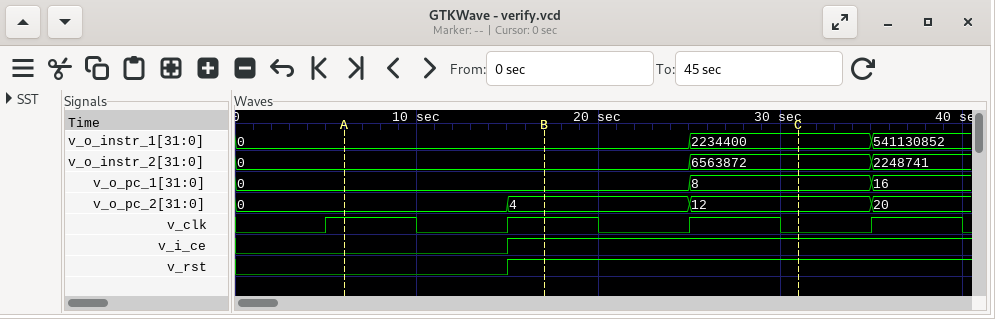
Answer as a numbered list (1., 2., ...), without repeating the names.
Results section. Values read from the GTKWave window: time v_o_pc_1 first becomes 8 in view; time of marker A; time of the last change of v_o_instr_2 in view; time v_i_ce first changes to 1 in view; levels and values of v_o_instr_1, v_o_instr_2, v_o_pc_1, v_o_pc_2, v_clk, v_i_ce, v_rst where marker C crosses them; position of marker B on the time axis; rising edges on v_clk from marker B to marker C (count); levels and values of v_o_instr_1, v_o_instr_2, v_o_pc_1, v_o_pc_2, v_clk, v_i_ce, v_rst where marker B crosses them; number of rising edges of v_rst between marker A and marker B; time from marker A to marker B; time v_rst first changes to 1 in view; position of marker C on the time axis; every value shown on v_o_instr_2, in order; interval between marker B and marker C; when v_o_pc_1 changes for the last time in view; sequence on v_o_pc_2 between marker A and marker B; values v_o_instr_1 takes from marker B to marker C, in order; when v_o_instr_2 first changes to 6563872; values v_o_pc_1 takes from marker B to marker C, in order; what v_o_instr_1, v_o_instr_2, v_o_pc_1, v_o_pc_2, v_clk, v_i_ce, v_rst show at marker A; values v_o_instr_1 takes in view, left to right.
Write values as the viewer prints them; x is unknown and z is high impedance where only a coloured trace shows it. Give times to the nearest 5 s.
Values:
1. 25 s
2. 5 s
3. 35 s
4. 15 s
5. v_o_instr_1=2234400, v_o_instr_2=6563872, v_o_pc_1=8, v_o_pc_2=12, v_clk=0, v_i_ce=1, v_rst=1
6. 15 s
7. 1
8. v_o_instr_1=0, v_o_instr_2=0, v_o_pc_1=0, v_o_pc_2=4, v_clk=1, v_i_ce=1, v_rst=1
9. 1
10. 10 s
11. 15 s
12. 30 s
13. 0, 6563872, 2248741
14. 15 s
15. 35 s
16. 0, 4
17. 0, 2234400
18. 25 s
19. 0, 8
20. v_o_instr_1=0, v_o_instr_2=0, v_o_pc_1=0, v_o_pc_2=0, v_clk=1, v_i_ce=0, v_rst=0
21. 0, 2234400, 541130852
